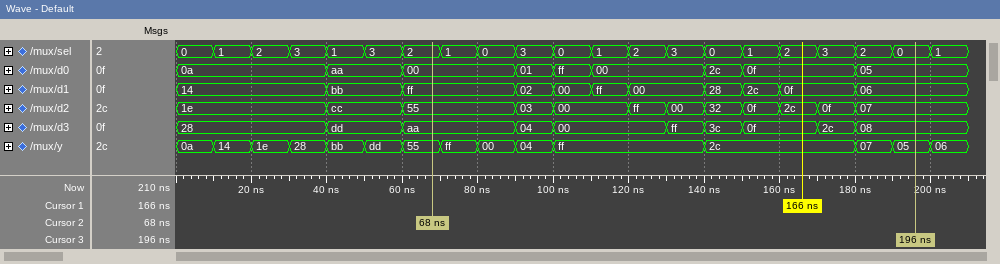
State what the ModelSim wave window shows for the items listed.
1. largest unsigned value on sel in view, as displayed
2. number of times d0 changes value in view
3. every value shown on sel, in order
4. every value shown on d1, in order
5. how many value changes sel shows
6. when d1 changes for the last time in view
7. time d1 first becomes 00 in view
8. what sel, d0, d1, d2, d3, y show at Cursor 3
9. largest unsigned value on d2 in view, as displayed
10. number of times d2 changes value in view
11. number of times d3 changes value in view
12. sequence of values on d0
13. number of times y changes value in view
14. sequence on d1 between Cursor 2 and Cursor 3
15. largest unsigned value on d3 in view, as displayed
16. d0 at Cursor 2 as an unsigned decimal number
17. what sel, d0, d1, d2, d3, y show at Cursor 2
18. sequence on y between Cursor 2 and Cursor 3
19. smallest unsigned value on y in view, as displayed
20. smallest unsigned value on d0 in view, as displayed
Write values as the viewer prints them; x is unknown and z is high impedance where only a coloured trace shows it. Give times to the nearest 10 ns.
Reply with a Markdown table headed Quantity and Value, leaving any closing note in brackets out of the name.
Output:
| Quantity | Value |
|---|---|
| largest unsigned value on sel in view, as displayed | 3 |
| number of times d0 changes value in view | 8 |
| every value shown on sel, in order | 0, 1, 2, 3, 1, 3, 2, 1, 0, 3, 0, 1, 2, 3, 0, 1, 2, 3, 2, 0, 1 |
| every value shown on d1, in order | 14, bb, ff, 02, 00, ff, 00, 28, 2c, 0f, 06 |
| how many value changes sel shows | 20 |
| when d1 changes for the last time in view | 180 ns |
| time d1 first becomes 00 in view | 100 ns |
| what sel, d0, d1, d2, d3, y show at Cursor 3 | sel=0, d0=05, d1=06, d2=07, d3=08, y=05 |
| largest unsigned value on d2 in view, as displayed | ff |
| number of times d2 changes value in view | 11 |
| number of times d3 changes value in view | 9 |
| sequence of values on d0 | 0a, aa, 00, 01, ff, 00, 2c, 0f, 05 |
| number of times y changes value in view | 14 |
| sequence on d1 between Cursor 2 and Cursor 3 | ff, 02, 00, ff, 00, 28, 2c, 0f, 06 |
| largest unsigned value on d3 in view, as displayed | ff |
| d0 at Cursor 2 as an unsigned decimal number | 0 |
| what sel, d0, d1, d2, d3, y show at Cursor 2 | sel=2, d0=00, d1=ff, d2=55, d3=aa, y=55 |
| sequence on y between Cursor 2 and Cursor 3 | 55, ff, 00, 04, ff, 2c, 07, 05 |
| smallest unsigned value on y in view, as displayed | 00 |
| smallest unsigned value on d0 in view, as displayed | 00 |
